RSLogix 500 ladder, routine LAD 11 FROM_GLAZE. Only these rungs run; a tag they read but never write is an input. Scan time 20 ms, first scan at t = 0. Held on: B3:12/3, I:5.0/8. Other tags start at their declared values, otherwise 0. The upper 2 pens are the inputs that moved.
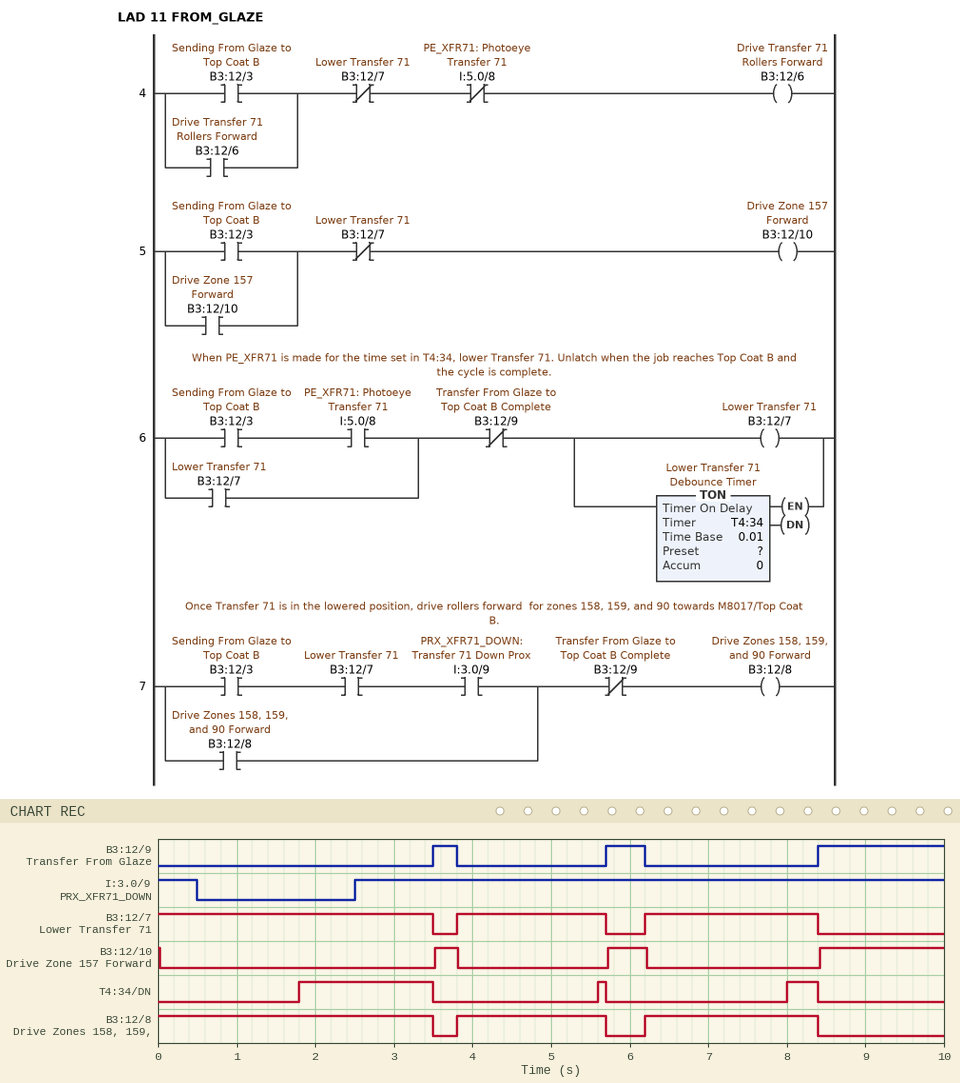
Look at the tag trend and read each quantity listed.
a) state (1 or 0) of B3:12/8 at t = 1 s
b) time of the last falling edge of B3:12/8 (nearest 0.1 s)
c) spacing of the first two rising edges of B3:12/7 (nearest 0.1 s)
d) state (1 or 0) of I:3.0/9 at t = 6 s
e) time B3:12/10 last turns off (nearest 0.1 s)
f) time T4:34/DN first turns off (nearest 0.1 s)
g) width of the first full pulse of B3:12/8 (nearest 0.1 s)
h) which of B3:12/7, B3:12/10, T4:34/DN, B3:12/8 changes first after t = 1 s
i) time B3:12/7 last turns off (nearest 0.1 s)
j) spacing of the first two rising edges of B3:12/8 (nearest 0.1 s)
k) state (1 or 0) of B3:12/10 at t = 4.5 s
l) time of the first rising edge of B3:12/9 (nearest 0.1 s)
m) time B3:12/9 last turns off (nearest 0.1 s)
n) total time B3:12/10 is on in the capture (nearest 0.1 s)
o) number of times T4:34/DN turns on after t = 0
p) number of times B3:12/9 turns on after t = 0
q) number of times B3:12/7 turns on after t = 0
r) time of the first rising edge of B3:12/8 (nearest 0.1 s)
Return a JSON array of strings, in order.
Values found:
["1", "8.4 s", "2.4 s", "1", "6.2 s", "3.5 s", "1.9 s", "T4:34/DN", "8.4 s", "2.4 s", "0", "3.5 s", "6.2 s", "2.4 s", "3", "3", "2", "3.8 s"]
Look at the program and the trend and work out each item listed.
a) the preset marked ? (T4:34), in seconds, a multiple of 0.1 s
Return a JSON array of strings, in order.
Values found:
["1.8 s"]
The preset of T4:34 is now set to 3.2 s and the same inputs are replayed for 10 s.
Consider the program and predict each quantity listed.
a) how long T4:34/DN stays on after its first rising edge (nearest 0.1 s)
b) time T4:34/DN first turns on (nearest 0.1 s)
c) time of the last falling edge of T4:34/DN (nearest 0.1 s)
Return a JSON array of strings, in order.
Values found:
["0.3 s", "3.2 s", "3.5 s"]
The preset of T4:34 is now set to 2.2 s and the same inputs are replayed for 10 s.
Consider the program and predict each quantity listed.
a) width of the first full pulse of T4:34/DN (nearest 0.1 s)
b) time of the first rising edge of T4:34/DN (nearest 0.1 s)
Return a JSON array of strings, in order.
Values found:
["1.3 s", "2.2 s"]
